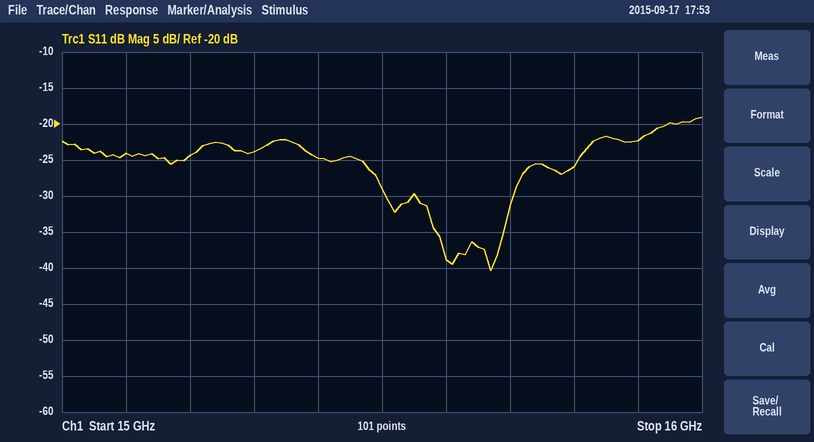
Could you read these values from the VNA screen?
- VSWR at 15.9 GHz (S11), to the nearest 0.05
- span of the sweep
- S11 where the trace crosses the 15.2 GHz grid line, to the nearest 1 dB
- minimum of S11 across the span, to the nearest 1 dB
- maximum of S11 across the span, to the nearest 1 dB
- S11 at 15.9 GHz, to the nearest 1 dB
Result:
1.15
1 GHz
-24 dB
-40 dB
-19 dB
-22 dB
